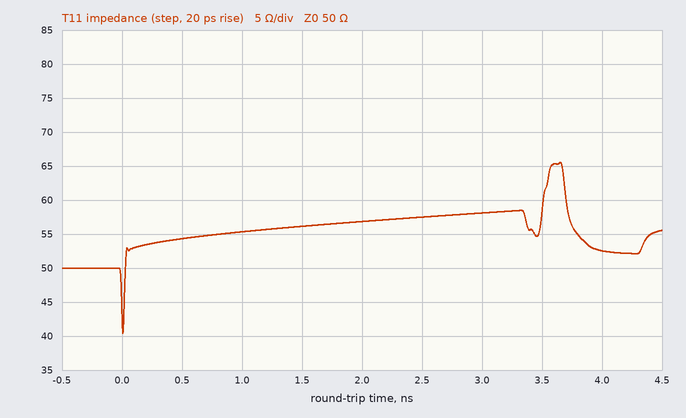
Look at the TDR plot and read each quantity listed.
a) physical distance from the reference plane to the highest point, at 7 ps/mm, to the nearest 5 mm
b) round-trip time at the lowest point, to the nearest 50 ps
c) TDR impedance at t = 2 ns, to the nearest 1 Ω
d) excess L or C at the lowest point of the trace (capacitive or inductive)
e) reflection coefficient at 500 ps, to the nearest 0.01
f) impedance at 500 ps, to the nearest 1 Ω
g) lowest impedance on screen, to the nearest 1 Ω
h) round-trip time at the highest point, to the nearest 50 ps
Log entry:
260 mm
0 ps
57 Ω
capacitive
+0.04
54 Ω
40 Ω
3.65 ns
